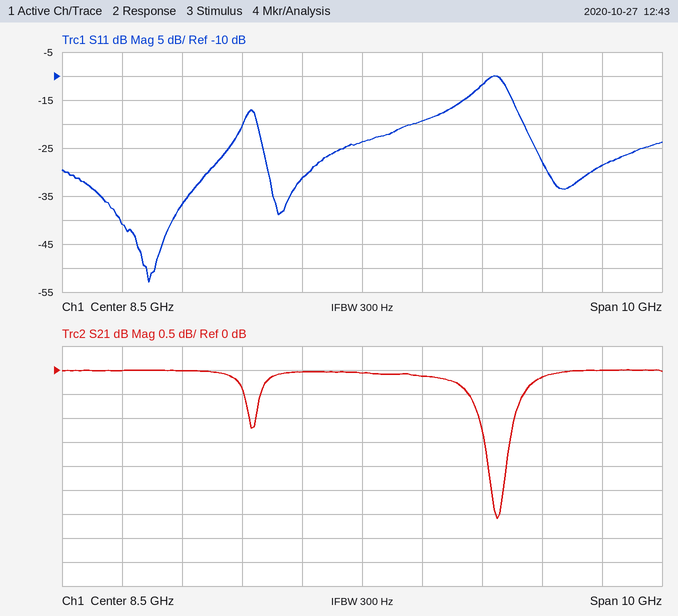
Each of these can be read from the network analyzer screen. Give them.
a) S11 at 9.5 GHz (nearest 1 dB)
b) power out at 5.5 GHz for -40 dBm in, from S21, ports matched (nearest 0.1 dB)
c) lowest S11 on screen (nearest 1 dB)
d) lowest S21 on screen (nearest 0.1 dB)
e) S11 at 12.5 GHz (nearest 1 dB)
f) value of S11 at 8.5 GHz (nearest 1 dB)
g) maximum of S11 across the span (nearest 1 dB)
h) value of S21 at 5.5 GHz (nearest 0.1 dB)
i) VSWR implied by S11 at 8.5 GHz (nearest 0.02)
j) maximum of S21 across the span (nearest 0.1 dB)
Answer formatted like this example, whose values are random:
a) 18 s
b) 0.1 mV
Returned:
a) -19 dB
b) -40.0 dBm
c) -53 dB
d) -3.1 dB
e) -29 dB
f) -24 dB
g) -10 dB
h) 0.0 dB
i) 1.14
j) 0.0 dB
